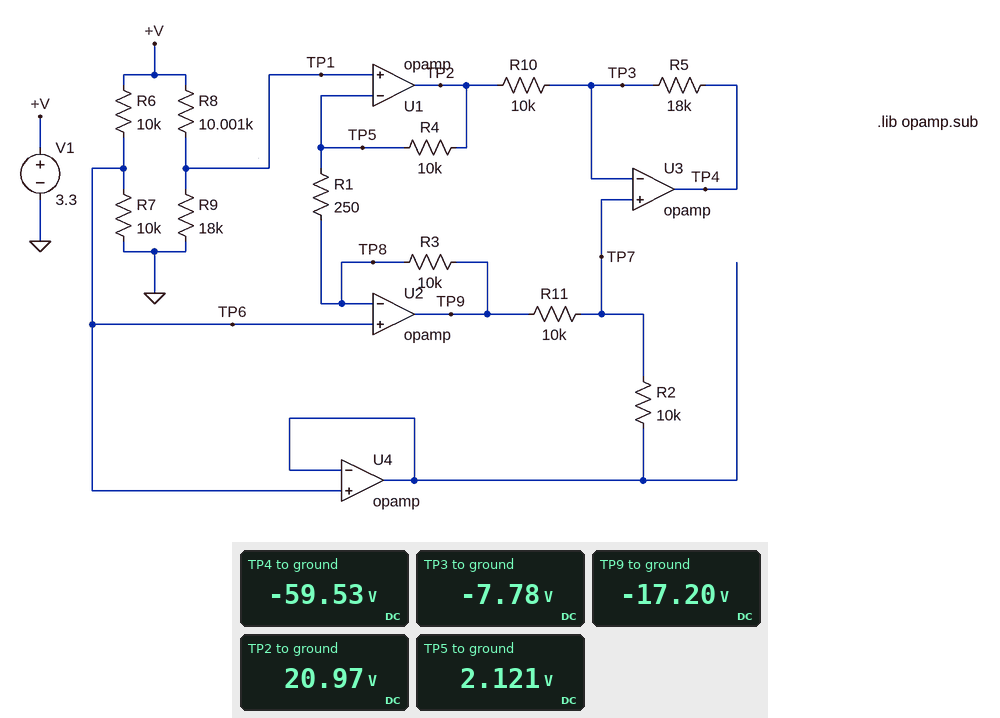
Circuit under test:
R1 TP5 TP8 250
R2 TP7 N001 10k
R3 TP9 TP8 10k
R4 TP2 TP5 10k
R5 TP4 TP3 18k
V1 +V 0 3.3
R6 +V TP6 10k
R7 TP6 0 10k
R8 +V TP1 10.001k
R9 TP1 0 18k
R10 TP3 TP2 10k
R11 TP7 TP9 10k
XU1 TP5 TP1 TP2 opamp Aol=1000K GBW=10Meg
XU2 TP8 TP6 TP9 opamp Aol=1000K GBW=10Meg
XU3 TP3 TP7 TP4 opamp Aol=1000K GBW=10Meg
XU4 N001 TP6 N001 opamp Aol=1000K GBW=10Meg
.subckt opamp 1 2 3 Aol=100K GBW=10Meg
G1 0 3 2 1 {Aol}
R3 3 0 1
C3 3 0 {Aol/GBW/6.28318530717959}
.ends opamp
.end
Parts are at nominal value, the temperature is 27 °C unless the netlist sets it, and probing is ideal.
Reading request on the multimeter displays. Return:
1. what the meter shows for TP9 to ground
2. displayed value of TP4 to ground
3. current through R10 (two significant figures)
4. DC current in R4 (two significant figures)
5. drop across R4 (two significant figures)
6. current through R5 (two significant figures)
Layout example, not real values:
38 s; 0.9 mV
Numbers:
-17.20 V; -59.53 V; 2.9 mA; 1.9 mA; 19 V; 2.9 mA
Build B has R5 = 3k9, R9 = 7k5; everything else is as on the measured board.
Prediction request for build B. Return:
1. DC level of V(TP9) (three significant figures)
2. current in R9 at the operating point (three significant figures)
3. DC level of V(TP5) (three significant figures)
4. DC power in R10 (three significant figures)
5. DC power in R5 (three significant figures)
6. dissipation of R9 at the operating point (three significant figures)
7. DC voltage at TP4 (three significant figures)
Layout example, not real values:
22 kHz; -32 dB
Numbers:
11.1 V; 189 µA; 1.41 V; 20.7 mW; 8.07 mW; 267 µW; 12.0 V
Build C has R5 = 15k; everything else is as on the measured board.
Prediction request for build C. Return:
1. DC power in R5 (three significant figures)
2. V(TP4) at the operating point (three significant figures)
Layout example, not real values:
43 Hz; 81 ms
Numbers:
124 mW; -50.9 V
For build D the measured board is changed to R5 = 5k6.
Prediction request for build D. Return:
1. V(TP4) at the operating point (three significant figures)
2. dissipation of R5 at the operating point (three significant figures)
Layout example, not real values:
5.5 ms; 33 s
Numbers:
-23.9 V; 46.3 mW
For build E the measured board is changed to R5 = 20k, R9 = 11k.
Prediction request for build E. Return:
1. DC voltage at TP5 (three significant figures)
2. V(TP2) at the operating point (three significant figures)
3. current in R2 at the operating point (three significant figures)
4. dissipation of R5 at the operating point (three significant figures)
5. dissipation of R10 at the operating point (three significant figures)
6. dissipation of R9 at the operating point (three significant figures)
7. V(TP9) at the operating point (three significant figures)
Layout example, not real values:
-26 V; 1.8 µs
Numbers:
1.73 V; 4.87 V; 157 µA; 4.58 mW; 2.29 mW; 272 µW; -1.49 V
